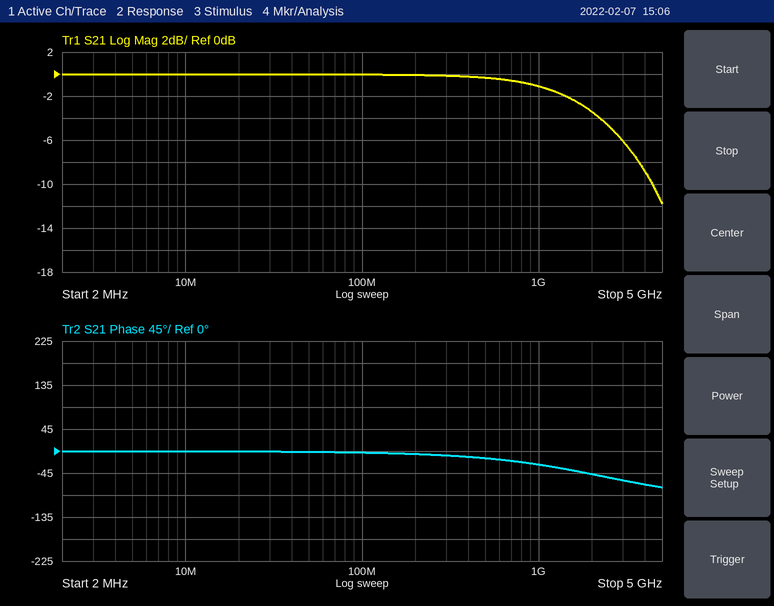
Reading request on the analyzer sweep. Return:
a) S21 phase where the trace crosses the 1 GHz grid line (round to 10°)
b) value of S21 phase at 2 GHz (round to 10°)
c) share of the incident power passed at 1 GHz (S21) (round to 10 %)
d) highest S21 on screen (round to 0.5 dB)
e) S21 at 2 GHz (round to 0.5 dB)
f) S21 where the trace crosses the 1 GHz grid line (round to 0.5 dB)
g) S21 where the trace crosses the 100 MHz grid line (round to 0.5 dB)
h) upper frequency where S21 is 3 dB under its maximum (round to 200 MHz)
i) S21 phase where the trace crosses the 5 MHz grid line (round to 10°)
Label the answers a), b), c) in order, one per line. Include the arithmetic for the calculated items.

a) -30°
b) -50°
c) 10^(-1/10) ≈ 79.4 %, so 80 % to the nearest 10 %
d) 0.0 dB
e) -3.5 dB
f) -1.0 dB
g) 0.0 dB
h) 1.8 GHz
i) 0°
